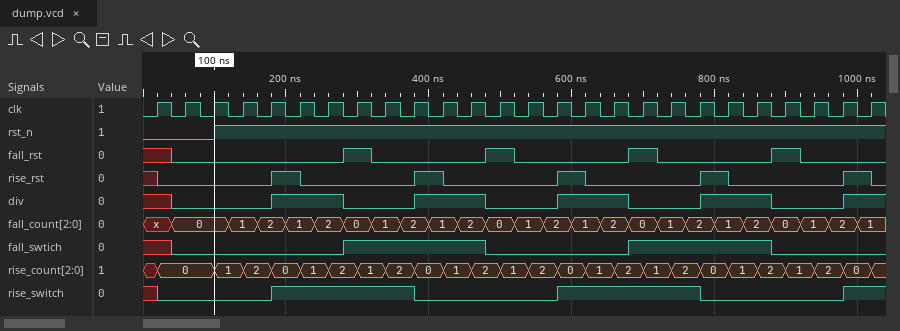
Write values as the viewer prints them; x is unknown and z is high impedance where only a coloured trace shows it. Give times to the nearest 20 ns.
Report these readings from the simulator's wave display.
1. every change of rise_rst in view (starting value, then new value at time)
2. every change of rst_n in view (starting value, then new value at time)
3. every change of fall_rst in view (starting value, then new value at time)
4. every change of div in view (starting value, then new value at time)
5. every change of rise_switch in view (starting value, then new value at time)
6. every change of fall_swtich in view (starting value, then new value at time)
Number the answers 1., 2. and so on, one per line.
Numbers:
1. x, 0 at 20 ns, 1 at 180 ns, 0 at 220 ns, 1 at 380 ns, 0 at 420 ns, 1 at 580 ns, 0 at 620 ns, 1 at 780 ns, 0 at 820 ns, 1 at 980 ns, 0 at 1020 ns
2. 0, 1 at 100 ns
3. x, 0 at 40 ns, 1 at 280 ns, 0 at 320 ns, 1 at 480 ns, 0 at 520 ns, 1 at 680 ns, 0 at 720 ns, 1 at 880 ns, 0 at 920 ns
4. x, 0 at 40 ns, 1 at 180 ns, 0 at 280 ns, 1 at 380 ns, 0 at 480 ns, 1 at 580 ns, 0 at 680 ns, 1 at 780 ns, 0 at 880 ns, 1 at 980 ns
5. x, 0 at 20 ns, 1 at 180 ns, 0 at 380 ns, 1 at 580 ns, 0 at 780 ns, 1 at 980 ns
6. x, 0 at 40 ns, 1 at 280 ns, 0 at 480 ns, 1 at 680 ns, 0 at 880 ns
